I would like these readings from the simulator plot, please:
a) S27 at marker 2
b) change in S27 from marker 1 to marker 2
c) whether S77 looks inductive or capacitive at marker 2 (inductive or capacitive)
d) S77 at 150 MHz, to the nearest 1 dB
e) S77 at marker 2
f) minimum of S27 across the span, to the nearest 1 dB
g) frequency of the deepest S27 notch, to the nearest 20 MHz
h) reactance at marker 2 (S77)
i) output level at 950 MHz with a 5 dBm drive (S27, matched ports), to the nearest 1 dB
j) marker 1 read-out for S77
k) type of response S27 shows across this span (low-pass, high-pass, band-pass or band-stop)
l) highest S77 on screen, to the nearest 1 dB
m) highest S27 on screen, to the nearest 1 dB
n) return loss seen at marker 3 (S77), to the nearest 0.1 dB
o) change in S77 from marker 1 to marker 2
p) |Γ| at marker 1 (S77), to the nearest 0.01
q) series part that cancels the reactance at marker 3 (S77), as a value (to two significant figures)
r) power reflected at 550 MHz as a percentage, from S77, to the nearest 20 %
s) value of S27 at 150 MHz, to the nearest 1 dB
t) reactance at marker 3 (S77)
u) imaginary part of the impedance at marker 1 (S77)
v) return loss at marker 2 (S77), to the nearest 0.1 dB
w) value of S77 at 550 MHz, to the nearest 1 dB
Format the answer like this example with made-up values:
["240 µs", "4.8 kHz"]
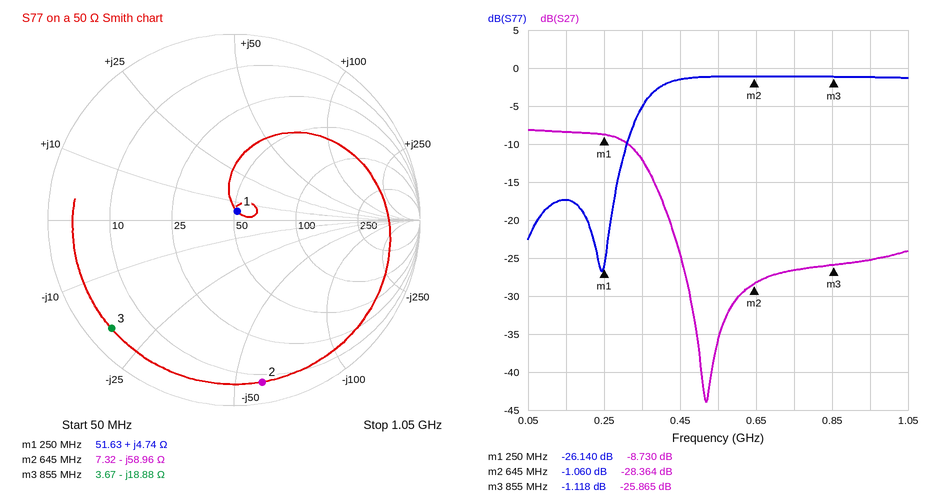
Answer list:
["-28.364 dB", "-19.634 dB", "capacitive", "-17 dB", "-1.060 dB", "-44 dB", "520 MHz", "-58.96 Ω", "-20 dBm", "-26.140 dB", "low-pass", "-1 dB", "-8 dB", "1.1 dB", "25.080 dB", "0.05", "3.5 nH", "80 %", "-8 dB", "-18.88 Ω", "+4.74 Ω", "1.1 dB", "-1 dB"]
